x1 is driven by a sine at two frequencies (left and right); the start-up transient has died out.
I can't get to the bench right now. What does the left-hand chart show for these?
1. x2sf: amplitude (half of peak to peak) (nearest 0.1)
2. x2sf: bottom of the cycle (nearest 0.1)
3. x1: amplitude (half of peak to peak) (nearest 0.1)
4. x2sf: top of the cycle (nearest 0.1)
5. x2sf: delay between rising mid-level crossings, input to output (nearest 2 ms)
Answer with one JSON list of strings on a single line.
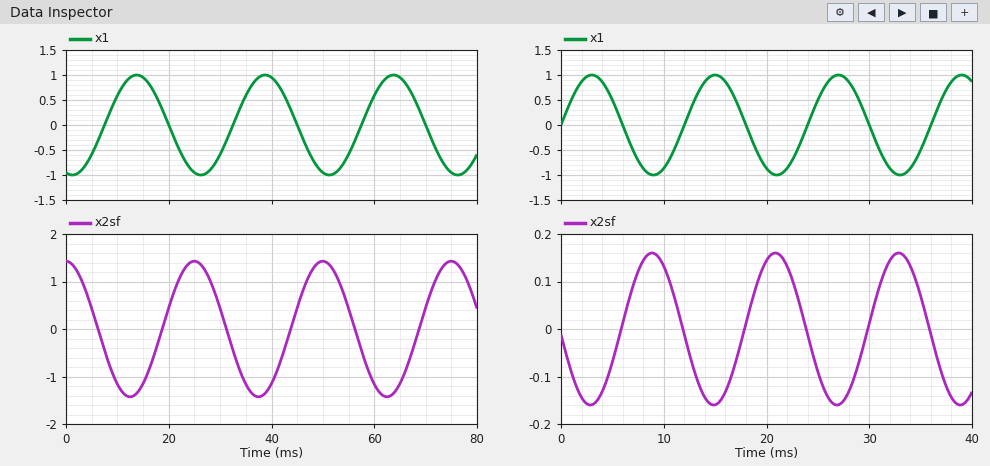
["1.4", "-1.4", "1.0", "1.4", "12 ms"]
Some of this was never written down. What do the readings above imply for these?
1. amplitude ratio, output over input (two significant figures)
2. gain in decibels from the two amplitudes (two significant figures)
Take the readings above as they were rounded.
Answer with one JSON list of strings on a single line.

["1.4", "2.9 dB"]
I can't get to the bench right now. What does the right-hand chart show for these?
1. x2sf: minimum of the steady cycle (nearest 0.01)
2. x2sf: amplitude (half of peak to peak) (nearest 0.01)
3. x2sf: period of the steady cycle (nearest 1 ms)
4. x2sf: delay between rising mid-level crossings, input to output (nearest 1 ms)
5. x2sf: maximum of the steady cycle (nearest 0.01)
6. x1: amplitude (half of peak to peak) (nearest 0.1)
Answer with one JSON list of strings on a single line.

["-0.16", "0.16", "12 ms", "6 ms", "0.16", "1.0"]
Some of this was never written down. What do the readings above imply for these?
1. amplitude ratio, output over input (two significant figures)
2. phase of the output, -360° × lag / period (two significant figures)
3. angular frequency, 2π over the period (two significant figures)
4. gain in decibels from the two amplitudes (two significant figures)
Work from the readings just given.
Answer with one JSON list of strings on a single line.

["0.16", "-180°", "0.52 rad/ms", "-16 dB"]
